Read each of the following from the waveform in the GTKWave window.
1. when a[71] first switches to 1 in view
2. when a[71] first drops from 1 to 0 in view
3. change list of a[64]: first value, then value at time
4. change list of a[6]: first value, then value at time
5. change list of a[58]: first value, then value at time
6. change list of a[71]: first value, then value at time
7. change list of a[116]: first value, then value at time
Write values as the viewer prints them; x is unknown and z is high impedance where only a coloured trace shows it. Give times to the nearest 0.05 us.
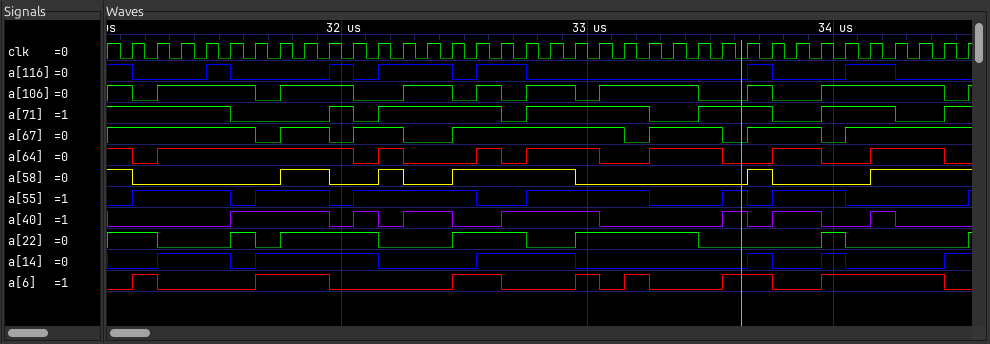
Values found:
31.95 us
31.55 us
1, 0 at 31.15 us, 1 at 31.25 us, 0 at 32.05 us, 1 at 32.15 us, 0 at 32.25 us, 1 at 32.55 us, 0 at 32.65 us, 1 at 32.75 us, 0 at 33.05 us, 1 at 33.25 us, 0 at 33.55 us, 1 at 33.75 us, 0 at 33.95 us, 1 at 34.15 us, 0 at 34.45 us
0, 1 at 31.15 us, 0 at 31.25 us, 1 at 31.65 us, 0 at 31.95 us, 1 at 32.45 us, 0 at 32.65 us, 1 at 32.95 us, 0 at 33.05 us, 1 at 33.15 us, 0 at 33.25 us, 1 at 33.55 us, 0 at 33.75 us, 1 at 33.95 us, 0 at 34.45 us
1, 0 at 31.15 us, 1 at 31.75 us, 0 at 31.95 us, 1 at 32.15 us, 0 at 32.25 us, 1 at 32.45 us, 0 at 32.95 us, 1 at 33.65 us, 0 at 33.75 us, 1 at 34.15 us
1, 0 at 31.55 us, 1 at 31.95 us, 0 at 32.05 us, 1 at 32.15 us, 0 at 32.65 us, 1 at 32.75 us, 0 at 33.25 us, 1 at 33.45 us, 0 at 33.75 us, 1 at 33.95 us, 0 at 34.25 us, 1 at 34.45 us
1, 0 at 31.15 us, 1 at 31.45 us, 0 at 31.55 us, 1 at 31.95 us, 0 at 32.05 us, 1 at 32.15 us, 0 at 32.45 us, 1 at 32.55 us, 0 at 32.75 us, 1 at 33.65 us, 0 at 33.75 us, 1 at 34.05 us, 0 at 34.25 us
